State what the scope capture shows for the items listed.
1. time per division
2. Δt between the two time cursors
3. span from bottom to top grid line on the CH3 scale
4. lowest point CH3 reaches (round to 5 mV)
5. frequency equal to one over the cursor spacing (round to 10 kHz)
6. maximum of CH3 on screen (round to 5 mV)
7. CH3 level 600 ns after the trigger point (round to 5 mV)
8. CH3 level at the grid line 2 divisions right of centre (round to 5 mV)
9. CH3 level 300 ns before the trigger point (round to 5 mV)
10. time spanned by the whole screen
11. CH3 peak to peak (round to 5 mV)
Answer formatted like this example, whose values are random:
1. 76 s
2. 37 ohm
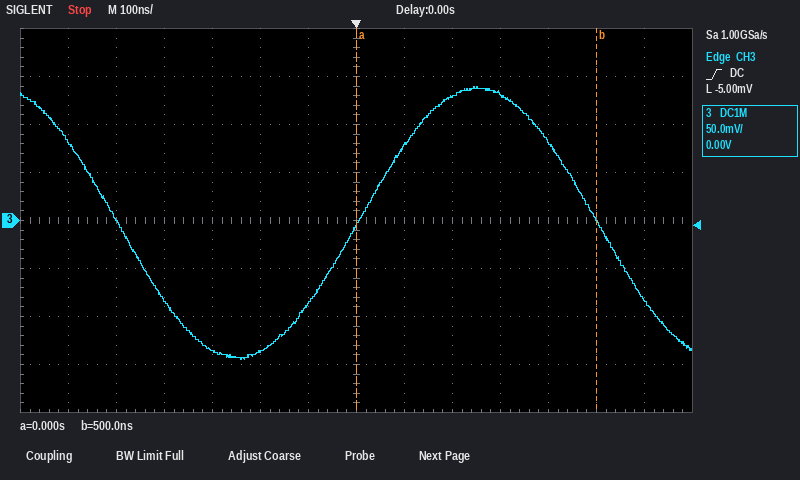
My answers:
1. 100 ns
2. 500 ns
3. 400 mV
4. -145 mV
5. 2.00 MHz
6. 140 mV
7. -80 mV
8. 130 mV
9. -135 mV
10. 1.4 µs
11. 285 mV
